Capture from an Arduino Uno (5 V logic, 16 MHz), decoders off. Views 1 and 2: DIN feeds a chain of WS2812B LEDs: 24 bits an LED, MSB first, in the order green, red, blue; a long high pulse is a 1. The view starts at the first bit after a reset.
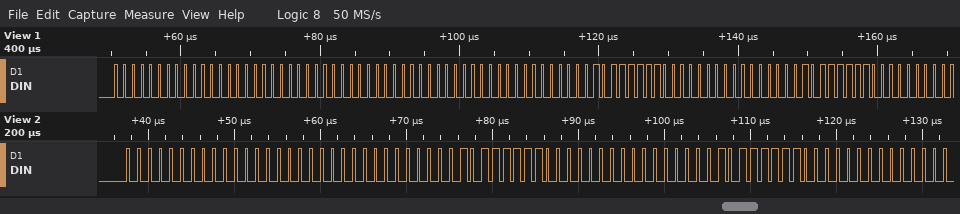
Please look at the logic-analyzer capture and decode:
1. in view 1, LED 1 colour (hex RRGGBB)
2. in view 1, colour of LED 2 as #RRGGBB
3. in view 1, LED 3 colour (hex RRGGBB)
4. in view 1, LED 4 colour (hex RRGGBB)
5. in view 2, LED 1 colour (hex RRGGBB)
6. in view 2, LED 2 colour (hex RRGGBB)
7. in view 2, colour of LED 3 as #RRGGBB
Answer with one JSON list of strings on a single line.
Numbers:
["#000000", "#000000", "#7E0100", "#7E0100", "#000000", "#7E0100", "#7E0100"]
